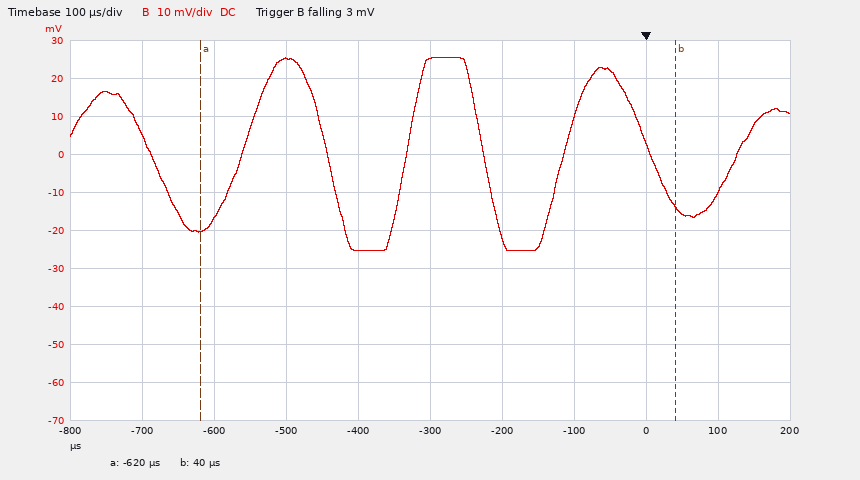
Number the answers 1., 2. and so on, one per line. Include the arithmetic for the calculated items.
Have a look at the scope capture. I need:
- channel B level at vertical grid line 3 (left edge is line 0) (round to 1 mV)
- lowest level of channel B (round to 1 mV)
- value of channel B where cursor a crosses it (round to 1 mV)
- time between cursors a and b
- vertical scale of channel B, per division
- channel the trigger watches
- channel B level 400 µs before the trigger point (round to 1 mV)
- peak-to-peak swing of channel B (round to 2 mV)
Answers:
1. 25 mV
2. -25 mV
3. -20 mV
4. 40 µs − (-620 µs) = 660 µs
5. 10 mV
6. channel B
7. -25 mV
8. 50 mV
